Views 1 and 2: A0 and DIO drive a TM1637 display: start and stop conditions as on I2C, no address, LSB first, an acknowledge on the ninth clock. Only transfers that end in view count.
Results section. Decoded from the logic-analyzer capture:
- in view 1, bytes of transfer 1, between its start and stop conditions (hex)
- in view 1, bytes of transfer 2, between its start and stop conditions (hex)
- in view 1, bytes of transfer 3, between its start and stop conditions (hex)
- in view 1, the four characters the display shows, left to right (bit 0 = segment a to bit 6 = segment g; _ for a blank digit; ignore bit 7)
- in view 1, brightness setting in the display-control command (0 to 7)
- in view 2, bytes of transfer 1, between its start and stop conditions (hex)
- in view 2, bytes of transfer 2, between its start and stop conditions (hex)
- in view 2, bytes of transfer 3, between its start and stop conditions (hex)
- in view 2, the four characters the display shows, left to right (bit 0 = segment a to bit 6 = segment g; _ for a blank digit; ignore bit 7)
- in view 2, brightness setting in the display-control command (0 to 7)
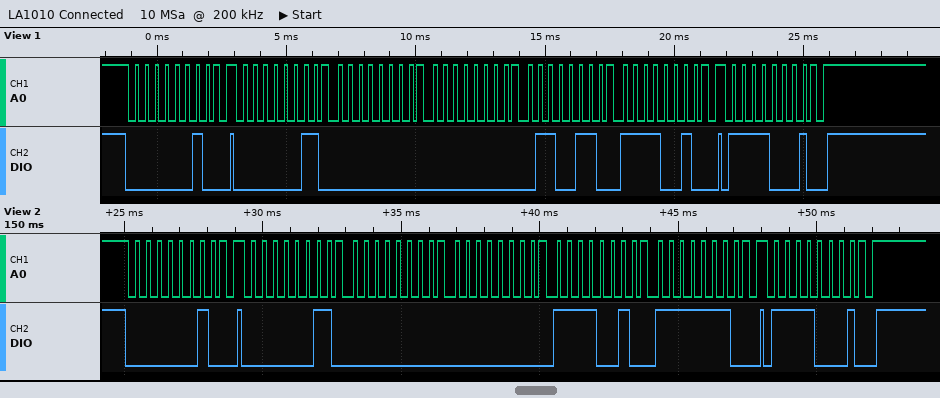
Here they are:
40
C0 00 00 66 4F
8F
__43
7
40
C0 00 00 4F 7F
8F
__38
7
